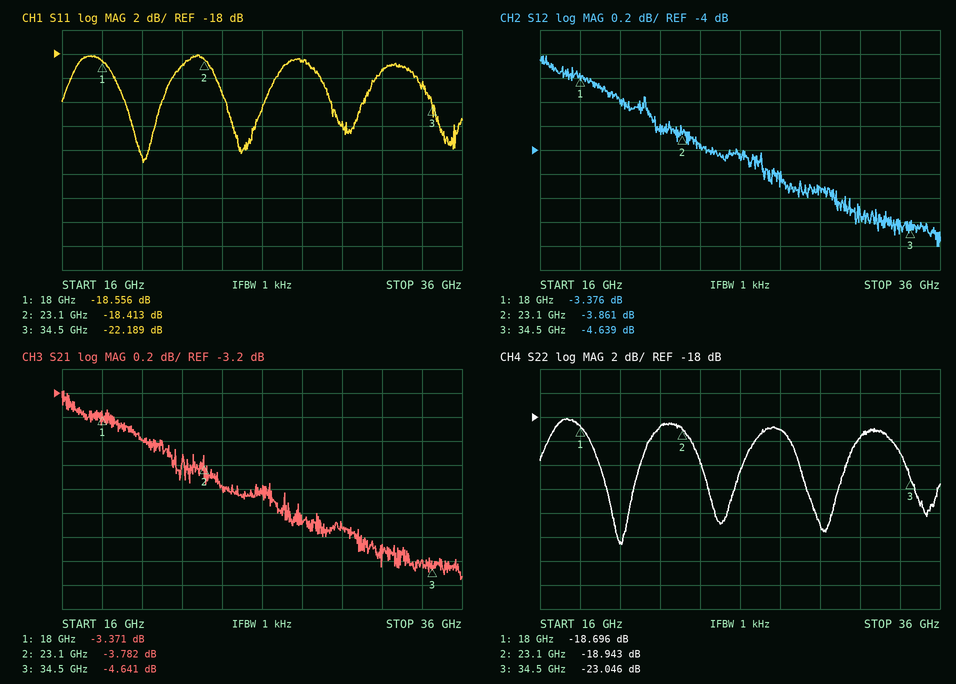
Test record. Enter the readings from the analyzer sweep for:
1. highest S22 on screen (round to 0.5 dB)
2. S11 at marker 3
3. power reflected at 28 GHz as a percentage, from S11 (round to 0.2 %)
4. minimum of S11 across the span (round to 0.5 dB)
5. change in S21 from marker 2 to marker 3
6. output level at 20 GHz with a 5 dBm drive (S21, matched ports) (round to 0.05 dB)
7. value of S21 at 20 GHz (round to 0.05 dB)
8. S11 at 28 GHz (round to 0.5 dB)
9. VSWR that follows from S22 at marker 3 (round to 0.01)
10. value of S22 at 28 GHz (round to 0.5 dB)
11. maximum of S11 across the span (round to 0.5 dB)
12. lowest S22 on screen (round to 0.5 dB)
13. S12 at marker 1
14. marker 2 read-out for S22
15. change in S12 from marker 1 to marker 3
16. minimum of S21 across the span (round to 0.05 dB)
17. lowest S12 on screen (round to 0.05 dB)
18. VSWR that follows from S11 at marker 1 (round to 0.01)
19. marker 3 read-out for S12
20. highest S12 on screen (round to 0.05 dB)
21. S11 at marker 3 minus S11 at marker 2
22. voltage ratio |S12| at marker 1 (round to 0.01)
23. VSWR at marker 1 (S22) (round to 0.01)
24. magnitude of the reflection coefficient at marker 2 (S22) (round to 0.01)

-18.0 dB
-22.189 dB
1.4 %
-27.0 dB
-0.859 dB
1.40 dBm
-3.60 dB
-18.5 dB
1.15
-19.0 dB
-18.0 dB
-28.5 dB
-3.376 dB
-18.943 dB
-1.263 dB
-4.75 dB
-4.80 dB
1.27
-4.639 dB
-3.20 dB
-3.776 dB
0.68
1.26
0.11
